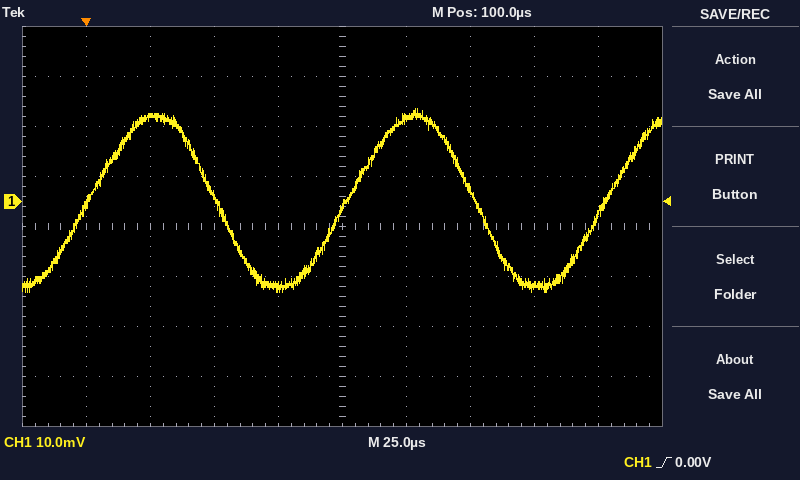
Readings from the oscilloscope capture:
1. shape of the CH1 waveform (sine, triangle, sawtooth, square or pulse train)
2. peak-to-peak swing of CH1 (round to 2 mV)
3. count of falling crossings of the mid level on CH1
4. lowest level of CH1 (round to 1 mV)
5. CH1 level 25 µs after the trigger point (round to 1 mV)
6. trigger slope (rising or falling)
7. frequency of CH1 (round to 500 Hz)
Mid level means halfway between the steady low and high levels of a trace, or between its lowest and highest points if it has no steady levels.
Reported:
sine
36 mV
2
-18 mV
17 mV
rising
10.0 kHz
